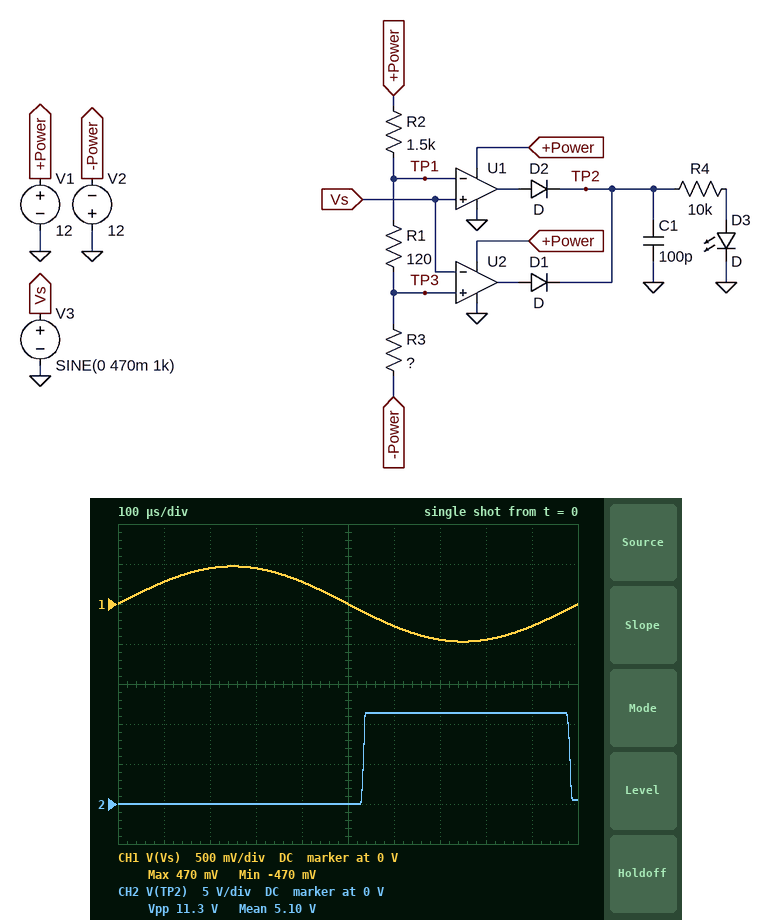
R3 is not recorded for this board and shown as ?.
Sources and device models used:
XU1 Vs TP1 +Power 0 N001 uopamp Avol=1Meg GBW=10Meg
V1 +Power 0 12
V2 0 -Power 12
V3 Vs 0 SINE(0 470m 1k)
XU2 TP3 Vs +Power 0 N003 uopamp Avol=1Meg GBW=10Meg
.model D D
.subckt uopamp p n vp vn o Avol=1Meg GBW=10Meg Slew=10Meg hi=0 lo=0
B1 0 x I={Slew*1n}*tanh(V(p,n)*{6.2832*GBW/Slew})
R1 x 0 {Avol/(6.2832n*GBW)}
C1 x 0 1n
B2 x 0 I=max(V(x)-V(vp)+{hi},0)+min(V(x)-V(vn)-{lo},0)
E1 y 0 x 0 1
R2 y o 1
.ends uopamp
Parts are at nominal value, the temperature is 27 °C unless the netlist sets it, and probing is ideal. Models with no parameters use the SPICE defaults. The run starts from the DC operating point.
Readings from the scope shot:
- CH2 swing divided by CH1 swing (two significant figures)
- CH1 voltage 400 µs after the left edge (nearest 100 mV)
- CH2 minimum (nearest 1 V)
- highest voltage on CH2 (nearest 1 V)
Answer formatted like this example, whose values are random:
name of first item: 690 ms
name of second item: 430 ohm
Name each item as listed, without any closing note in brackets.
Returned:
CH2 swing divided by CH1 swing: 12
CH1 voltage 400 µs after the left edge: 300 mV
CH2 minimum: 0 V
highest voltage on CH2: 11 V
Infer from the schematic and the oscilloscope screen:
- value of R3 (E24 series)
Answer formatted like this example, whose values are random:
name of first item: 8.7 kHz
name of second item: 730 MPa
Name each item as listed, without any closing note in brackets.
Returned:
value of R3: 1.6 kΩ
